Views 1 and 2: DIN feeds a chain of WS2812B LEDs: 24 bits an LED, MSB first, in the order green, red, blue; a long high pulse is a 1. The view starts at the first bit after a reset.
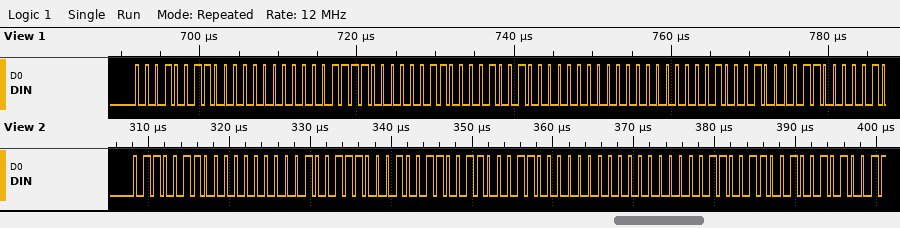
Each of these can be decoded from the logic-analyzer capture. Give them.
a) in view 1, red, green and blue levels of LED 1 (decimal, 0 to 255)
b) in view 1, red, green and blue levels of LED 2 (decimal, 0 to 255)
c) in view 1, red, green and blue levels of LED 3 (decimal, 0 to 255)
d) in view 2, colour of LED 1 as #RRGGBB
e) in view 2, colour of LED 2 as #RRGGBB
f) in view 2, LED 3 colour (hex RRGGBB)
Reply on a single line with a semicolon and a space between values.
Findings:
0, 19, 15; 9, 3, 0; 17, 0, 12; #00664E; #632600; #66004A
